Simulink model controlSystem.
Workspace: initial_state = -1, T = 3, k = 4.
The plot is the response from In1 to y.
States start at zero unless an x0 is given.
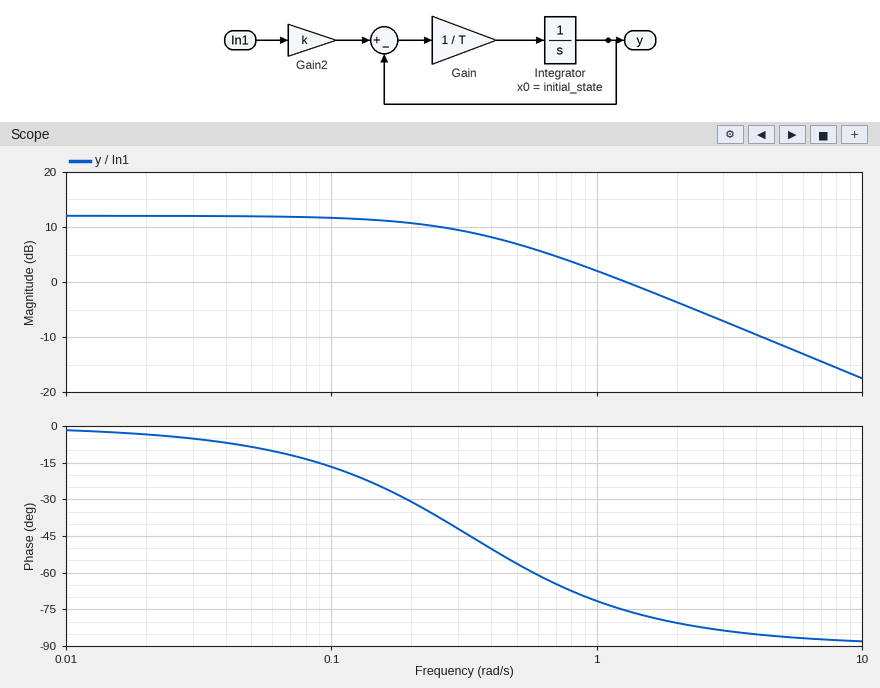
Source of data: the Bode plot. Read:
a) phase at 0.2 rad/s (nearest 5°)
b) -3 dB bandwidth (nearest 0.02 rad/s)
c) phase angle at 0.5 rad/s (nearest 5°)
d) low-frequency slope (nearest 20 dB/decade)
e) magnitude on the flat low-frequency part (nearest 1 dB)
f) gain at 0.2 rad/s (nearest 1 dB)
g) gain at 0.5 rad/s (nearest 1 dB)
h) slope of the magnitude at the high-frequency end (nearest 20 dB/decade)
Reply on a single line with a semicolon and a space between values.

-30°; 0.34 rad/s; -55°; 0 dB/decade; 12 dB; 11 dB; 7 dB; -20 dB/decade
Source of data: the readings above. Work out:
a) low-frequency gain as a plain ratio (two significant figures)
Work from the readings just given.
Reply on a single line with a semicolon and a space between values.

4.0
